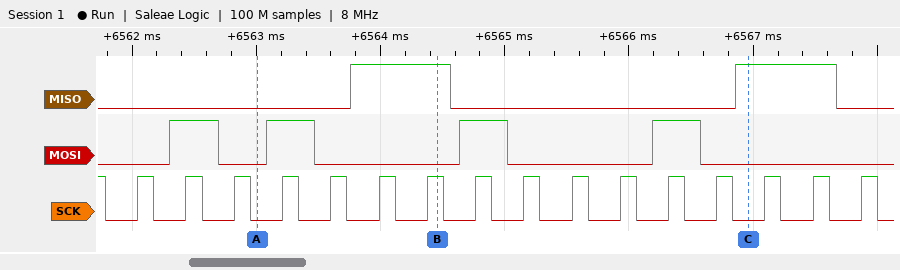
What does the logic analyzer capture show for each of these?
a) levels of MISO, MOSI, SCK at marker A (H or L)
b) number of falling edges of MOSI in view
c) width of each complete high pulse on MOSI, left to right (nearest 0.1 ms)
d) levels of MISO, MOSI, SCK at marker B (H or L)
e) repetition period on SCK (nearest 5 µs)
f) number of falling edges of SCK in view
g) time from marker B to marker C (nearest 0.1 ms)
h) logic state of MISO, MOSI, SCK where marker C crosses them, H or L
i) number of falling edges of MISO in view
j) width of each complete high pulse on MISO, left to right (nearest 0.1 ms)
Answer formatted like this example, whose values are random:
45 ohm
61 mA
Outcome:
MISO=L, MOSI=L, SCK=L
4
0.4 ms, 0.4 ms, 0.4 ms, 0.4 ms
MISO=H, MOSI=L, SCK=H
390 µs
17
2.5 ms
MISO=H, MOSI=L, SCK=L
2
0.8 ms, 0.8 ms
